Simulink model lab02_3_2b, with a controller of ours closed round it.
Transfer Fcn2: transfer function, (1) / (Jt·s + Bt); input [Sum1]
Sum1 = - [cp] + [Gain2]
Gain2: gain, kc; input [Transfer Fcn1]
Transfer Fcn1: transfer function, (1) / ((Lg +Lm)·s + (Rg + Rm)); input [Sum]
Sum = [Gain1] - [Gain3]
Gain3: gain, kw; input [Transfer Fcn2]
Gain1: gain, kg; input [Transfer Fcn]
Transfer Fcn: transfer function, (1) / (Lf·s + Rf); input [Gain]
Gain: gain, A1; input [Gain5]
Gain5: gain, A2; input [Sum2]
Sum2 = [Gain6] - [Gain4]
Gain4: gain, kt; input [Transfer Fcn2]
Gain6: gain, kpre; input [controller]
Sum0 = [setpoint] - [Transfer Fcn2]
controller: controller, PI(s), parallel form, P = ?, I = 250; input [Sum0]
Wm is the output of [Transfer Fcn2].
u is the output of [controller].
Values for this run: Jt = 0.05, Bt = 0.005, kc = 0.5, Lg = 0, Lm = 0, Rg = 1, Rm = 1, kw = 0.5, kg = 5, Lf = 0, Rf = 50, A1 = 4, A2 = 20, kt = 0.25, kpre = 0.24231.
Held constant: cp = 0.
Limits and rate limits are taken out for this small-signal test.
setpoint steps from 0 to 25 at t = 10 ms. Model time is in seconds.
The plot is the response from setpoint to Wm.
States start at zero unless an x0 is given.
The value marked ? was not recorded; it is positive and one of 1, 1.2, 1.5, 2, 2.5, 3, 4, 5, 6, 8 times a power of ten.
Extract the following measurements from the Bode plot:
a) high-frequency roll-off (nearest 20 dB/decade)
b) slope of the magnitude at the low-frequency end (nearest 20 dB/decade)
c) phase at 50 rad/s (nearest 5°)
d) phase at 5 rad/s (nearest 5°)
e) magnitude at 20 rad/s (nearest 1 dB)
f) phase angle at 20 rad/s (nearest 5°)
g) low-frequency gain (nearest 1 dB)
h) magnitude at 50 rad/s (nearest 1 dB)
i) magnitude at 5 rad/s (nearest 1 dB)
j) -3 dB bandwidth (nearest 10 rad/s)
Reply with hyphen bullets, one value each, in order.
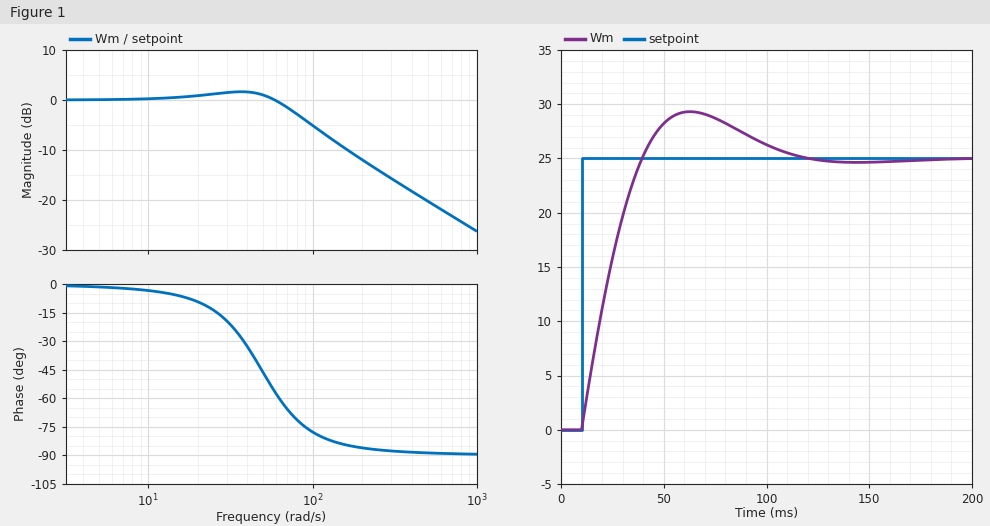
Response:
- -20 dB/decade
- 0 dB/decade
- -45°
- 0°
- 1 dB
- -10°
- 0 dB
- 1 dB
- 0 dB
- 80 rad/s
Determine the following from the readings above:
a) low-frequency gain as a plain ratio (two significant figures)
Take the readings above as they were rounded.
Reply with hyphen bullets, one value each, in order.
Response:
- 1.0
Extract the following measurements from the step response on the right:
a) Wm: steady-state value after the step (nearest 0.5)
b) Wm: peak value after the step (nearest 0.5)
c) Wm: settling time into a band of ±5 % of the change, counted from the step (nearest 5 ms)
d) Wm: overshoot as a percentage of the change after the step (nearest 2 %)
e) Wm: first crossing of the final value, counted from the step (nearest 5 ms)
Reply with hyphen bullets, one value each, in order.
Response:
- 25.0
- 29.5
- 90 ms
- 18 %
- 30 ms
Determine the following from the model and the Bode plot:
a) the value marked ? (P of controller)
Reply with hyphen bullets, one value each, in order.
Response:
- 5
